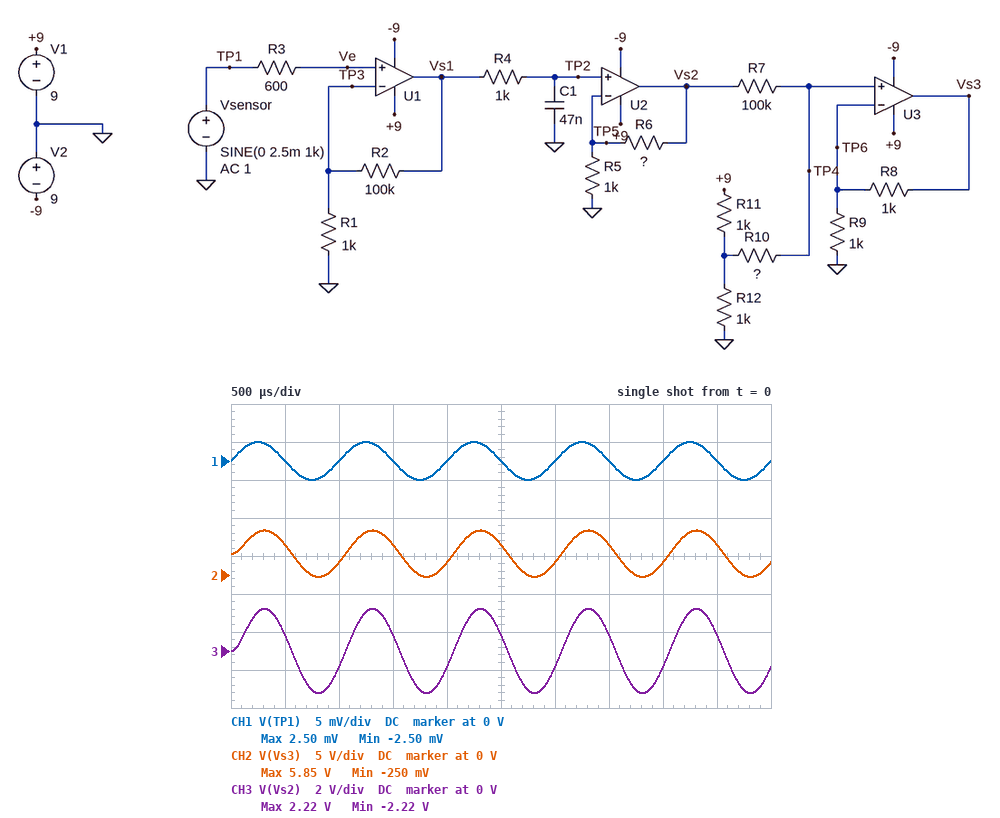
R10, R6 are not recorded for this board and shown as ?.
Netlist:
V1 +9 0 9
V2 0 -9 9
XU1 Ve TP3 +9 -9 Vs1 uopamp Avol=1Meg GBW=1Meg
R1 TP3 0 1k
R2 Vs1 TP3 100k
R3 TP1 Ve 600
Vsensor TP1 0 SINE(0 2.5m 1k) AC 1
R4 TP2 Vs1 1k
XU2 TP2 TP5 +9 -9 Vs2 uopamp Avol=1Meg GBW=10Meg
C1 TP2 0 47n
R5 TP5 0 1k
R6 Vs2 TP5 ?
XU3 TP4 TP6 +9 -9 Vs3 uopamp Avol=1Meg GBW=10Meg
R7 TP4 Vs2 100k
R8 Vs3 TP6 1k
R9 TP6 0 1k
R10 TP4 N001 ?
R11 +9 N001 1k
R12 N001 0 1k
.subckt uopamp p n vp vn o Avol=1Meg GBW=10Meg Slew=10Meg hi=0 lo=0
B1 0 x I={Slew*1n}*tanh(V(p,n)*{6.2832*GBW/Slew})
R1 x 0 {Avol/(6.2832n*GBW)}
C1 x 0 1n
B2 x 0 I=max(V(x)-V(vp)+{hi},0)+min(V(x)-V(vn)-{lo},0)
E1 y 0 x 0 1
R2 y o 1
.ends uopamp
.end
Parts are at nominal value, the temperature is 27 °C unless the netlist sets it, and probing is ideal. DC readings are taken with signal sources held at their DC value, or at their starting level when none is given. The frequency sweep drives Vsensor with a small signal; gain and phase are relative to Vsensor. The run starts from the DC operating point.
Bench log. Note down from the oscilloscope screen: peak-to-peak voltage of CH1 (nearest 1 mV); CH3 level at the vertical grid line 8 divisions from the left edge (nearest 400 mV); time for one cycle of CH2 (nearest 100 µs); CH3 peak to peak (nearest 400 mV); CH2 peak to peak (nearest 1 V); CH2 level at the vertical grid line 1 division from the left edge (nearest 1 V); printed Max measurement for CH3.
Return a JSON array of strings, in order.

["5 mV", "-800 mV", "1.0 ms", "4.4 V", "6 V", "4 V", "2.22 V"]
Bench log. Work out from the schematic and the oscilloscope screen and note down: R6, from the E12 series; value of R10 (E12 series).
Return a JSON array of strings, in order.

["8.2 kΩ", "220 kΩ"]
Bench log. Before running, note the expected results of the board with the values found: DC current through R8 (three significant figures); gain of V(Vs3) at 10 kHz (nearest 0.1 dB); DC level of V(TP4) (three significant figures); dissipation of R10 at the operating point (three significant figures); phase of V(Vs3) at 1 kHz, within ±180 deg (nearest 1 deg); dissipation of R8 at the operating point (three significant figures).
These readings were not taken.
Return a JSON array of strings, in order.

["1.40 mA", "49.2 dB", "1.40 V", "43.4 µW", "-22 deg", "1.97 mW"]
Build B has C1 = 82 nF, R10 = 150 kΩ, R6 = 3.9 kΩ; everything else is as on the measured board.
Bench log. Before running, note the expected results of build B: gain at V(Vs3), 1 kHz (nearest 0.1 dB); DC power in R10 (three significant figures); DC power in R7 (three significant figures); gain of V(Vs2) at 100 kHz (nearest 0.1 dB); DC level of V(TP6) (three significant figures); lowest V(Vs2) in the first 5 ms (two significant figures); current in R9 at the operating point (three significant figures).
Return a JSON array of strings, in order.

["54.4 dB", "48.4 µW", "32.3 µW", "-0.5 dB", "1.80 V", "-1.1 V", "1.80 mA"]
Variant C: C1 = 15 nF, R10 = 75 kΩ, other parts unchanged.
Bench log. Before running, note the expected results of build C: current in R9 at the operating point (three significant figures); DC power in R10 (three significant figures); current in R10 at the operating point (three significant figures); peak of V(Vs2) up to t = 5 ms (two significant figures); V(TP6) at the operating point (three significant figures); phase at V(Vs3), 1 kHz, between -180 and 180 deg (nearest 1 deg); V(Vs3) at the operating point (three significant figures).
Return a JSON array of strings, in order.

["2.56 mA", "49.3 µW", "25.6 µA", "2.3 V", "2.56 V", "-11 deg", "5.13 V"]
